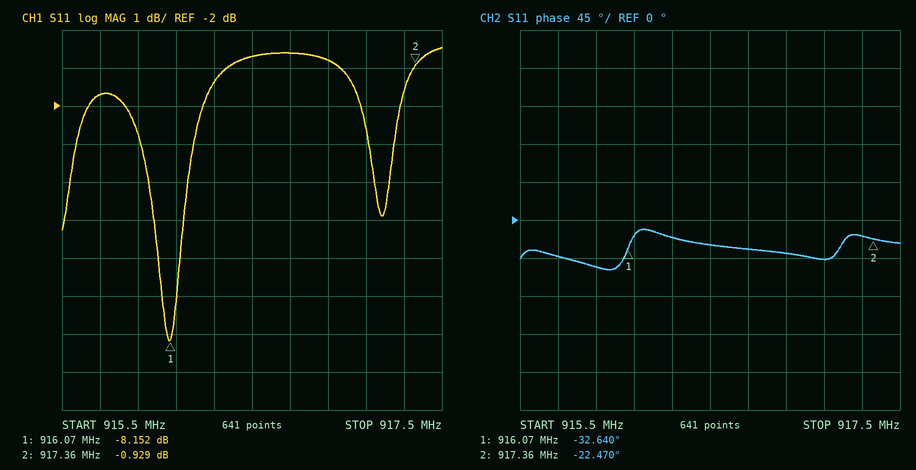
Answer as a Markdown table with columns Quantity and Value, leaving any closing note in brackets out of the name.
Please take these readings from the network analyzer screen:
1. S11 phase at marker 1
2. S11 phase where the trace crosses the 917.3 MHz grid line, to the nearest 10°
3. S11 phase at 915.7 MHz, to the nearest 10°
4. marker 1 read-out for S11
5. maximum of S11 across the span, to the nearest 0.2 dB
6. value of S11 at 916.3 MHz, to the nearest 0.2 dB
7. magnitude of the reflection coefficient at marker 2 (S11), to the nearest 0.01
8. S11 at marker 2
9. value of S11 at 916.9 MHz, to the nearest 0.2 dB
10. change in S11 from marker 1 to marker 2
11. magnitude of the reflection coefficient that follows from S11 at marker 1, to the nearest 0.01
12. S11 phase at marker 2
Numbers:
| Quantity | Value |
|---|---|
| S11 phase at marker 1 | -32.640° |
| S11 phase where the trace crosses the 917.3 MHz grid line, to the nearest 10° | -20° |
| S11 phase at 915.7 MHz, to the nearest 10° | -40° |
| marker 1 read-out for S11 | -8.152 dB |
| maximum of S11 across the span, to the nearest 0.2 dB | -0.4 dB |
| value of S11 at 916.3 MHz, to the nearest 0.2 dB | -1.4 dB |
| magnitude of the reflection coefficient at marker 2 (S11), to the nearest 0.01 | 0.90 |
| S11 at marker 2 | -0.929 dB |
| value of S11 at 916.9 MHz, to the nearest 0.2 dB | -0.8 dB |
| change in S11 from marker 1 to marker 2 | 7.223 dB |
| magnitude of the reflection coefficient that follows from S11 at marker 1, to the nearest 0.01 | 0.39 |
| S11 phase at marker 2 | -22.470° |
